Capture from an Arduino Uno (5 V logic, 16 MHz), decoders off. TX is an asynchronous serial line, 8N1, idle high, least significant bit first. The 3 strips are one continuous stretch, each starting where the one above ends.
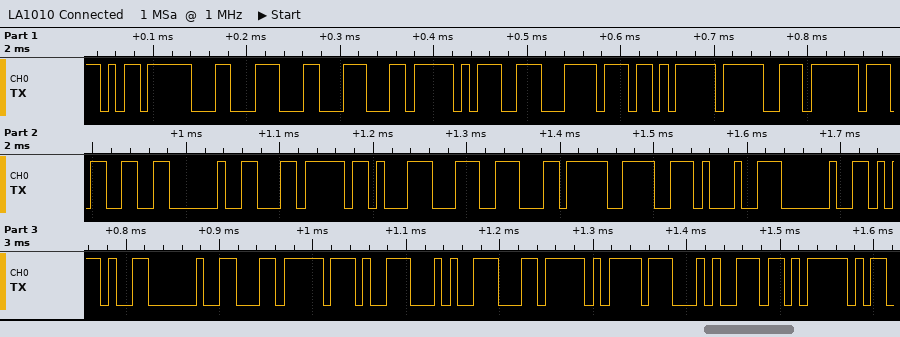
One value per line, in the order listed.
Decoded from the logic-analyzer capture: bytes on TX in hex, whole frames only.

ED 8C 8C EC 9D BC EB 9F BF 33 20 EC 8B 9C EC 9E 91 20 2D 20 EC 97 94 EC BD 94 EB
